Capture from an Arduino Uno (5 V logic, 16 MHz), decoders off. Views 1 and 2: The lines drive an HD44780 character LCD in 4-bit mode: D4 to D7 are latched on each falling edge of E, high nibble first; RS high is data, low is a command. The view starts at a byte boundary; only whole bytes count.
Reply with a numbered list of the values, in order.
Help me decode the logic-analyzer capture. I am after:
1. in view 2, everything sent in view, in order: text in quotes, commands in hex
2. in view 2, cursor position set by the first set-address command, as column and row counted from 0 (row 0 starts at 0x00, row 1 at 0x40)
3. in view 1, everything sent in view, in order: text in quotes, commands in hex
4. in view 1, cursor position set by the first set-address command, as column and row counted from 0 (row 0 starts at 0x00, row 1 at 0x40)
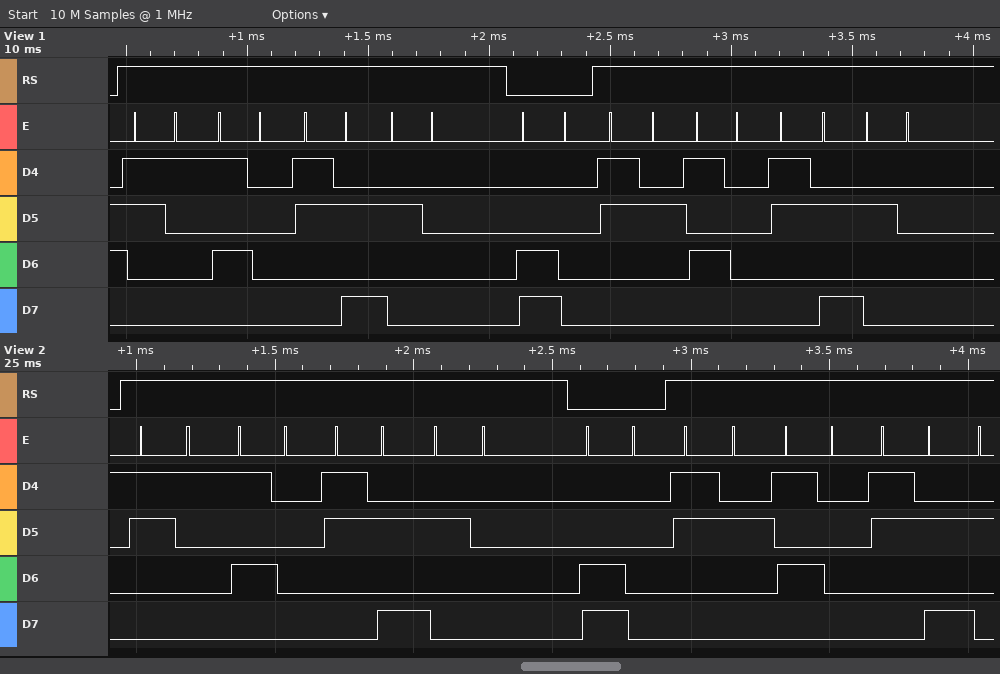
1. "1P: " 0xC0 "2P:"
2. column 0, row 1
3. "1P: " 0xC0 "2P: "
4. column 0, row 1
